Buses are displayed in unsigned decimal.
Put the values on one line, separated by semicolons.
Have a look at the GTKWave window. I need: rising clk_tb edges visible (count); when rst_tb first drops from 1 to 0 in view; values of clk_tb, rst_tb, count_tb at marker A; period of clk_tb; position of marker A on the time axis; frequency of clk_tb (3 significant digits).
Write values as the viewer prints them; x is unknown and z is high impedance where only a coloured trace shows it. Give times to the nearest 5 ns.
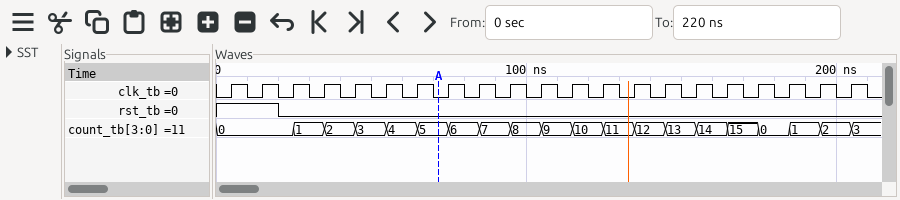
21; 20 ns; clk_tb=0, rst_tb=0, count_tb=5; 10 ns; 70 ns; 100 MHz
